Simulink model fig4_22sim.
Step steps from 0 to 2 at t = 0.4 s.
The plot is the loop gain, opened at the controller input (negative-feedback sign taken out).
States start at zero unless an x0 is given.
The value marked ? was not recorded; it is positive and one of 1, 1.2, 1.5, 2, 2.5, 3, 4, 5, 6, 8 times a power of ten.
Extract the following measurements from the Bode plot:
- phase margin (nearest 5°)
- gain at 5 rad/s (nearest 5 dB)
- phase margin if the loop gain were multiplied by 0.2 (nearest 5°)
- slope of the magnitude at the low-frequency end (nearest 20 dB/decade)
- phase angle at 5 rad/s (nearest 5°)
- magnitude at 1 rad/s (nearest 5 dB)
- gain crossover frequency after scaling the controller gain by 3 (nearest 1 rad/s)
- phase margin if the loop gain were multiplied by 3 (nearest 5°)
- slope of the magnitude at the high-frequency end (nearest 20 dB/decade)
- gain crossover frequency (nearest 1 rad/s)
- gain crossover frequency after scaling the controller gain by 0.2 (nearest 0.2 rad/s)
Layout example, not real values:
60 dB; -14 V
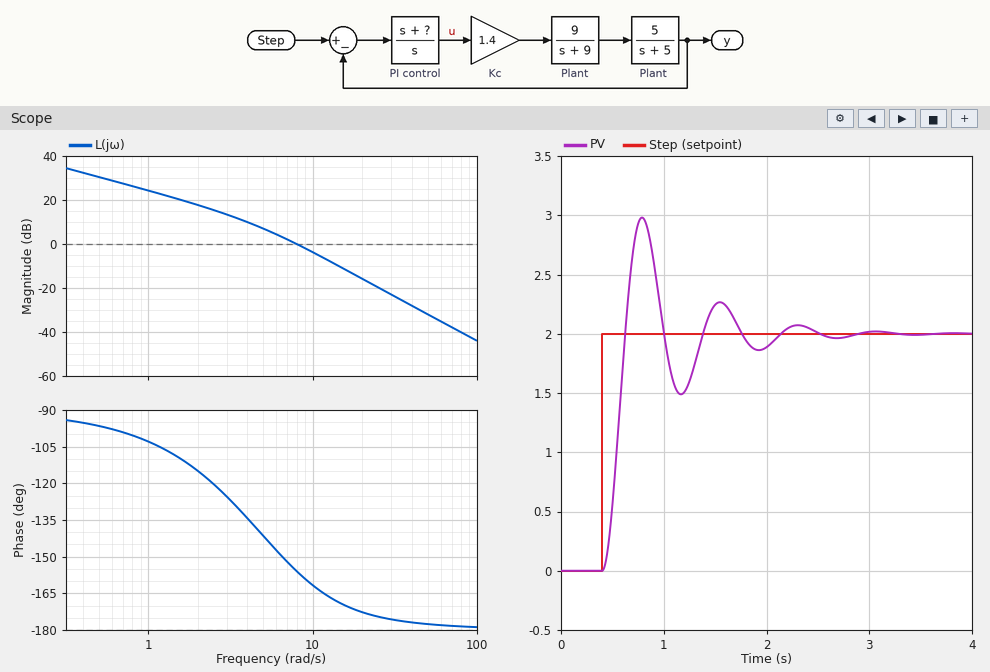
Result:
25°; 5 dB; 55°; -20 dB/decade; -140°; 25 dB; 14 rad/s; 10°; -40 dB/decade; 8 rad/s; 2.8 rad/s
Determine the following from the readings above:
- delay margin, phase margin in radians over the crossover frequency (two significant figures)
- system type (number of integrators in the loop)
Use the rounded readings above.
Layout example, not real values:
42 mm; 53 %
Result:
0.055 s; 1
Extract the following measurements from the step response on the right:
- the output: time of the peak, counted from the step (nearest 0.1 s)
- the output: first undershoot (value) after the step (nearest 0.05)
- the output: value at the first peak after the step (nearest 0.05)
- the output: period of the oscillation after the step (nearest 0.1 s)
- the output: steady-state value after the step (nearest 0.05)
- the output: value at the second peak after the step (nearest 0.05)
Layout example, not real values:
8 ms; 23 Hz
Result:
0.4 s; 1.50; 3.00; 0.8 s; 2.00; 2.25
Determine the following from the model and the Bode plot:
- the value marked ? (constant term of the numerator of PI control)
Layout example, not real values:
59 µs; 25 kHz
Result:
12
